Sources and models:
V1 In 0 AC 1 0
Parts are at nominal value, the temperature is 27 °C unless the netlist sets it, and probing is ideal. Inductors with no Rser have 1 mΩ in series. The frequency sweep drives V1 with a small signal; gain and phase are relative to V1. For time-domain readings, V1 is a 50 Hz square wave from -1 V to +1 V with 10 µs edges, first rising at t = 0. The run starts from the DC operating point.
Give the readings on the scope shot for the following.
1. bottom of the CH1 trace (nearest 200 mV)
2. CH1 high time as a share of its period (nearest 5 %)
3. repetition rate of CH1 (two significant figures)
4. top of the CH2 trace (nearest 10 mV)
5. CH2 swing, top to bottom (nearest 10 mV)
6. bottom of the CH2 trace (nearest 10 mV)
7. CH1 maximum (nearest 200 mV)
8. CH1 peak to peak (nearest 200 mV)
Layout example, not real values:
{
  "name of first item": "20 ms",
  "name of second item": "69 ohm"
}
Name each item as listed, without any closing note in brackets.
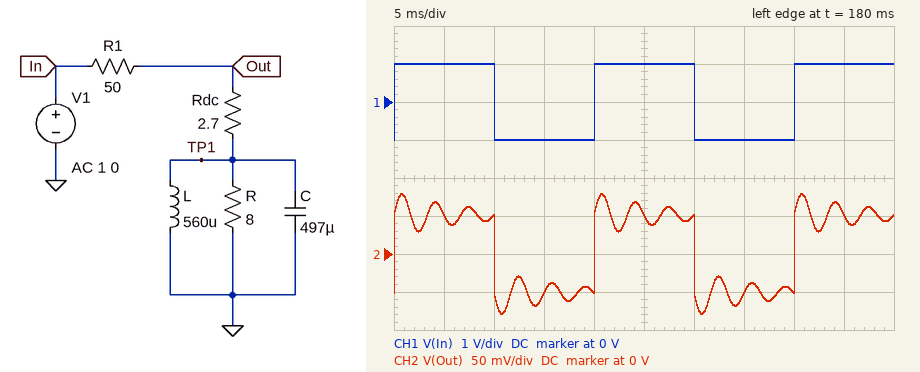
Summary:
{
  "bottom of the CH1 trace": "-1.0 V",
  "CH1 high time as a share of its period": "50 %",
  "repetition rate of CH1": "50 Hz",
  "top of the CH2 trace": "80 mV",
  "CH2 swing, top to bottom": "160 mV",
  "bottom of the CH2 trace": "-80 mV",
  "CH1 maximum": "1.0 V",
  "CH1 peak to peak": "2.0 V"
}
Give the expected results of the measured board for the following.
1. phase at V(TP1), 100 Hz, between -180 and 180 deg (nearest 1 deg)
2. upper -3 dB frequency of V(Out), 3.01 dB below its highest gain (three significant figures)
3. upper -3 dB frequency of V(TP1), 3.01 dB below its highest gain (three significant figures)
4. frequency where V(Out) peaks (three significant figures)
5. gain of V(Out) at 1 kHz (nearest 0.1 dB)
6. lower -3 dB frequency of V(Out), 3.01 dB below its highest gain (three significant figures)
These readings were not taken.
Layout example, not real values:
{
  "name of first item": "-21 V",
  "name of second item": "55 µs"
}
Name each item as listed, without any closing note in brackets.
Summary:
{
  "phase at V(TP1), 100 Hz, between -180 and 180 deg": "87 deg",
  "upper -3 dB frequency of V(Out), 3.01 dB below its highest gain": "328 Hz",
  "upper -3 dB frequency of V(TP1), 3.01 dB below its highest gain": "326 Hz",
  "frequency where V(Out) peaks": "302 Hz",
  "gain of V(Out) at 1 kHz": "-25.7 dB",
  "lower -3 dB frequency of V(Out), 3.01 dB below its highest gain": "277 Hz"
}
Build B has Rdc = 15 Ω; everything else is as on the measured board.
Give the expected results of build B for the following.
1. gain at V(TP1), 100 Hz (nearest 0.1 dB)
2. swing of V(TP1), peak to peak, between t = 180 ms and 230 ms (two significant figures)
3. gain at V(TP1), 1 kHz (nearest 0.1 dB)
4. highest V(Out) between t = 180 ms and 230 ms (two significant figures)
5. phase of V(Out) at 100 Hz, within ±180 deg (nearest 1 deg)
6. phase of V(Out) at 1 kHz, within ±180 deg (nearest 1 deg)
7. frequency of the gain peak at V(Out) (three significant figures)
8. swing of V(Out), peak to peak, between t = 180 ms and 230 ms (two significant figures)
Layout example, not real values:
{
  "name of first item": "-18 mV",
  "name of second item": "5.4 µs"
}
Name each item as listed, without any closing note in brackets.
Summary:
{
  "gain at V(TP1), 100 Hz": "-44.3 dB",
  "swing of V(TP1), peak to peak, between t = 180 ms and 230 ms": "47 mV",
  "gain at V(TP1), 1 kHz": "-45.3 dB",
  "highest V(Out) between t = 180 ms and 230 ms": "250 mV",
  "phase of V(Out) at 100 Hz, within ±180 deg": "1 deg",
  "phase of V(Out) at 1 kHz, within ±180 deg": "-1 deg",
  "frequency of the gain peak at V(Out)": "302 Hz",
  "swing of V(Out), peak to peak, between t = 180 ms and 230 ms": "500 mV"
}
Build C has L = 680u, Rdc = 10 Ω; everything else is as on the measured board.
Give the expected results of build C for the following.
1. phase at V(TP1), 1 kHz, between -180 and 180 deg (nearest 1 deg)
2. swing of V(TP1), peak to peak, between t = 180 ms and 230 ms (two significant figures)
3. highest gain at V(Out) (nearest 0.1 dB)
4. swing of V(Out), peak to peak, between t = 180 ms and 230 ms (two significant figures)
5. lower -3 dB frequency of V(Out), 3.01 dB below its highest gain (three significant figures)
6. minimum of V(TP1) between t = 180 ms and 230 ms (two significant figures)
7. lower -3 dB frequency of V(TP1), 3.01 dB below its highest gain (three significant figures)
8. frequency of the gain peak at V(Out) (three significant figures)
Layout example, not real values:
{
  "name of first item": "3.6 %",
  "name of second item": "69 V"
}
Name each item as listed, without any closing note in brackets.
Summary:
{
  "phase at V(TP1), 1 kHz, between -180 and 180 deg": "-87 deg",
  "swing of V(TP1), peak to peak, between t = 180 ms and 230 ms": "71 mV",
  "highest gain at V(Out)": "-11.6 dB",
  "swing of V(Out), peak to peak, between t = 180 ms and 230 ms": "390 mV",
  "lower -3 dB frequency of V(Out), 3.01 dB below its highest gain": "228 Hz",
  "minimum of V(TP1) between t = 180 ms and 230 ms": "-35 mV",
  "lower -3 dB frequency of V(TP1), 3.01 dB below its highest gain": "252 Hz",
  "frequency of the gain peak at V(Out)": "274 Hz"
}
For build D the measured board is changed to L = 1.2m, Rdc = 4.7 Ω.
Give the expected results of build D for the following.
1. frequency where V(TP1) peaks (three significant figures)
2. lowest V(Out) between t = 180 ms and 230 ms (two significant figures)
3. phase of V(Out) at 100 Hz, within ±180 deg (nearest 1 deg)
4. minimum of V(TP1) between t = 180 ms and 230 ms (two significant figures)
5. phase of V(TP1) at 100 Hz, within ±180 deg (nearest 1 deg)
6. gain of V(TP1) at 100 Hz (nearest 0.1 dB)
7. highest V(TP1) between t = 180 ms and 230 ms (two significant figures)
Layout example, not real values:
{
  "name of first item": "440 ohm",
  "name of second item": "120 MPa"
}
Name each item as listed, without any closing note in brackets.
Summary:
{
  "frequency where V(TP1) peaks": "206 Hz",
  "lowest V(Out) between t = 180 ms and 230 ms": "-120 mV",
  "phase of V(Out) at 100 Hz, within ±180 deg": "10 deg",
  "minimum of V(TP1) between t = 180 ms and 230 ms": "-39 mV",
  "phase of V(TP1) at 100 Hz, within ±180 deg": "82 deg",
  "gain of V(TP1) at 100 Hz": "-35.0 dB",
  "highest V(TP1) between t = 180 ms and 230 ms": "39 mV"
}
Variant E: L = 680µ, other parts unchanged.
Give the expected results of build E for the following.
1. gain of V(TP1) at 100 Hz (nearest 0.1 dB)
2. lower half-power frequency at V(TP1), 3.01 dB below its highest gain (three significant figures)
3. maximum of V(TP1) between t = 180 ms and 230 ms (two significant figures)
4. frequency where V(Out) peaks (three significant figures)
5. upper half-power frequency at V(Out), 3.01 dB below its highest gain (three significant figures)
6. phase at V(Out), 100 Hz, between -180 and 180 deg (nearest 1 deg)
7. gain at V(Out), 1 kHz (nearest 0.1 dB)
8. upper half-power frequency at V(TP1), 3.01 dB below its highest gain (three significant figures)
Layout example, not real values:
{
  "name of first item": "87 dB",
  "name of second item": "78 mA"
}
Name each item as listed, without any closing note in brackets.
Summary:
{
  "gain of V(TP1) at 100 Hz": "-40.6 dB",
  "lower half-power frequency at V(TP1), 3.01 dB below its highest gain": "252 Hz",
  "maximum of V(TP1) between t = 180 ms and 230 ms": "40 mV",
  "frequency where V(Out) peaks": "274 Hz",
  "upper half-power frequency at V(Out), 3.01 dB below its highest gain": "300 Hz",
  "phase at V(Out), 100 Hz, between -180 and 180 deg": "10 deg",
  "gain at V(Out), 1 kHz": "-25.7 dB",
  "upper half-power frequency at V(TP1), 3.01 dB below its highest gain": "298 Hz"
}
